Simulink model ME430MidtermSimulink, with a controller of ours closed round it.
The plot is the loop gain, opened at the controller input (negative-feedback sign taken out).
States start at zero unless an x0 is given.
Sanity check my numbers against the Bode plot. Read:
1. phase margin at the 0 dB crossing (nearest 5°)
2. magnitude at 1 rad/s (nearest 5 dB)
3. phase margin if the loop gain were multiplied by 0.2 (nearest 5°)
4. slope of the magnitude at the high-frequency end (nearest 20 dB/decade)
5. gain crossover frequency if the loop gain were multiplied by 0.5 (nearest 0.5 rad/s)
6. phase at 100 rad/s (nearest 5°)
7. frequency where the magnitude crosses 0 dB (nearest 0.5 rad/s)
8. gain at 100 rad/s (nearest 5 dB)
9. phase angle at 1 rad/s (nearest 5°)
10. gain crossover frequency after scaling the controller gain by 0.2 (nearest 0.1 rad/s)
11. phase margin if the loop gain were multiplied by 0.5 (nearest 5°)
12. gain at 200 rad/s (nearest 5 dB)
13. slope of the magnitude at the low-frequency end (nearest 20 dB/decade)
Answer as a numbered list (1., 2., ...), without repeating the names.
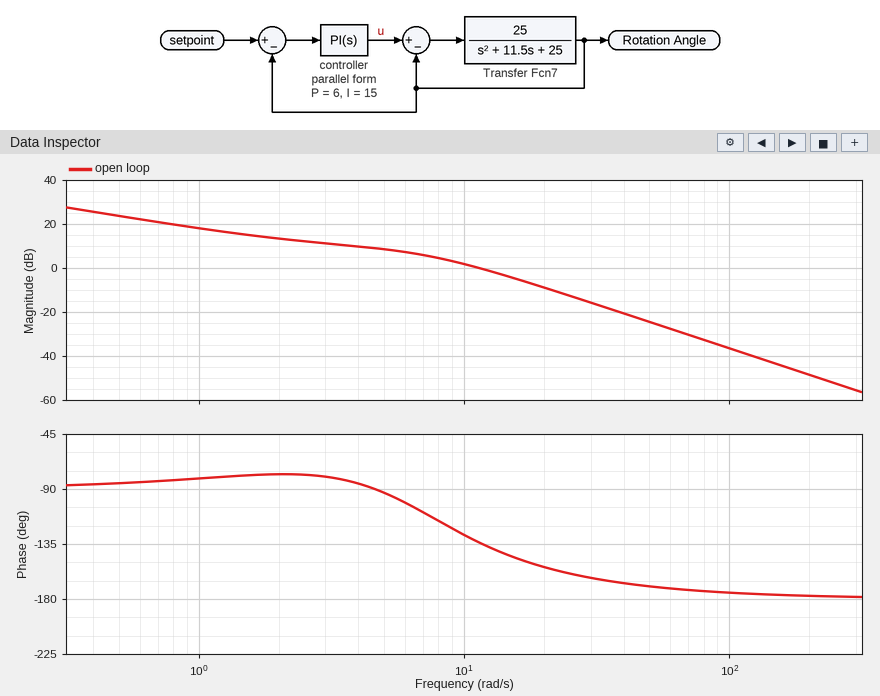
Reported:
1. 45°
2. 20 dB
3. 100°
4. -40 dB/decade
5. 7.0 rad/s
6. -175°
7. 11.5 rad/s
8. -35 dB
9. -80°
10. 1.8 rad/s
11. 70°
12. -50 dB
13. -20 dB/decade
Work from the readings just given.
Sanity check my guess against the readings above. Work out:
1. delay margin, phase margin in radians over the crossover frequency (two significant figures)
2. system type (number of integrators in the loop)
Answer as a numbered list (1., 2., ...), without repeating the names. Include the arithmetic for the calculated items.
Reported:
1. 45 × π / 180 / 11.5 = 0.068 s
2. 1
